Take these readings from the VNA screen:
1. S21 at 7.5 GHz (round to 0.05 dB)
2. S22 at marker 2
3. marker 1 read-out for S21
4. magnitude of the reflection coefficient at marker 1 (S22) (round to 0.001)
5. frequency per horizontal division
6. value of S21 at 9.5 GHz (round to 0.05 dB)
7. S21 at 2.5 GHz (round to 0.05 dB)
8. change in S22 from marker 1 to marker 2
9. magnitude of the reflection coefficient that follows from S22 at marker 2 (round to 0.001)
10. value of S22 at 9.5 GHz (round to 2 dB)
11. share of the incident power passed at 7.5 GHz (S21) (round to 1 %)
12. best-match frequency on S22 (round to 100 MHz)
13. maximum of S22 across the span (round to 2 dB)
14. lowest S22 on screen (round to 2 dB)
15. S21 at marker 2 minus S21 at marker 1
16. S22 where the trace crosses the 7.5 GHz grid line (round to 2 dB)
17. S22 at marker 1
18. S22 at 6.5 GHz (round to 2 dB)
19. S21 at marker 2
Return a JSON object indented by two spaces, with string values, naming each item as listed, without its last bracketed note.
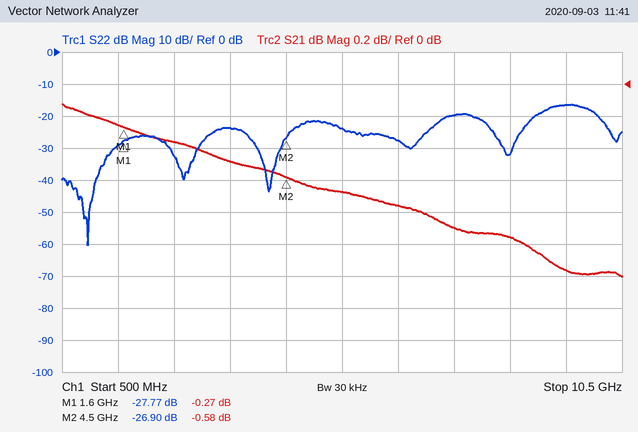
{
  "S21 at 7.5 GHz": "-0.90 dB",
  "S22 at marker 2": "-26.90 dB",
  "marker 1 read-out for S21": "-0.27 dB",
  "magnitude of the reflection coefficient at marker 1 (S22)": "0.041",
  "frequency per horizontal division": "1 GHz",
  "value of S21 at 9.5 GHz": "-1.15 dB",
  "S21 at 2.5 GHz": "-0.35 dB",
  "change in S22 from marker 1 to marker 2": "0.87 dB",
  "magnitude of the reflection coefficient that follows from S22 at marker 2": "0.045",
  "value of S22 at 9.5 GHz": "-16 dB",
  "share of the incident power passed at 7.5 GHz (S21)": "81 %",
  "best-match frequency on S22": "1.0 GHz",
  "maximum of S22 across the span": "-16 dB",
  "lowest S22 on screen": "-60 dB",
  "S21 at marker 2 minus S21 at marker 1": "-0.31 dB",
  "S22 where the trace crosses the 7.5 GHz grid line": "-20 dB",
  "S22 at marker 1": "-27.77 dB",
  "S22 at 6.5 GHz": "-28 dB",
  "S21 at marker 2": "-0.58 dB"
}
